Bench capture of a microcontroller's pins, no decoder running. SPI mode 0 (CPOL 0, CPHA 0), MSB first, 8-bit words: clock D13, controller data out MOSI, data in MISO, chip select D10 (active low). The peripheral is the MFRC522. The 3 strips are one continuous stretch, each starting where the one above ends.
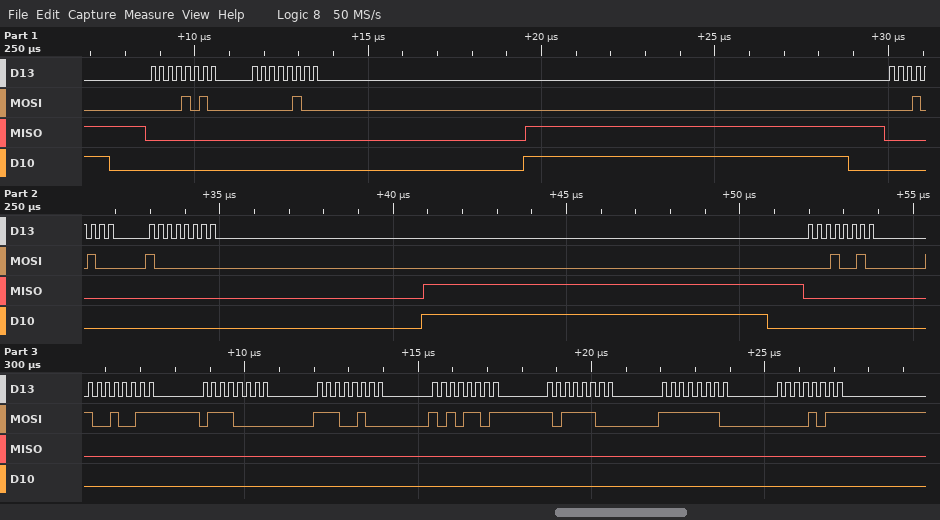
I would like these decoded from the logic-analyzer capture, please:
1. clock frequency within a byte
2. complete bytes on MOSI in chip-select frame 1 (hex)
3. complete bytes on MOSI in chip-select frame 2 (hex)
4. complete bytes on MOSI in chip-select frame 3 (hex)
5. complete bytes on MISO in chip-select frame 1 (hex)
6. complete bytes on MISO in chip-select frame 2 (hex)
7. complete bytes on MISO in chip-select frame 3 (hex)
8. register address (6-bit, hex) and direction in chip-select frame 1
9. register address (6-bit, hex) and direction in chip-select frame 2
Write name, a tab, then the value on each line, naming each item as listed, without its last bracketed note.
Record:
clock frequency within a byte	4 MHz
complete bytes on MOSI in chip-select frame 1	0A 04
complete bytes on MOSI in chip-select frame 2	14 80
complete bytes on MOSI in chip-select frame 3	12 93 70 E4 AD BC FE 0B
complete bytes on MISO in chip-select frame 1	00 00
complete bytes on MISO in chip-select frame 2	00 00
complete bytes on MISO in chip-select frame 3	00 00 00 00 00 00 00 00
register address (6-bit, hex) and direction in chip-select frame 1	0x05 write
register address (6-bit, hex) and direction in chip-select frame 2	0x0A write
